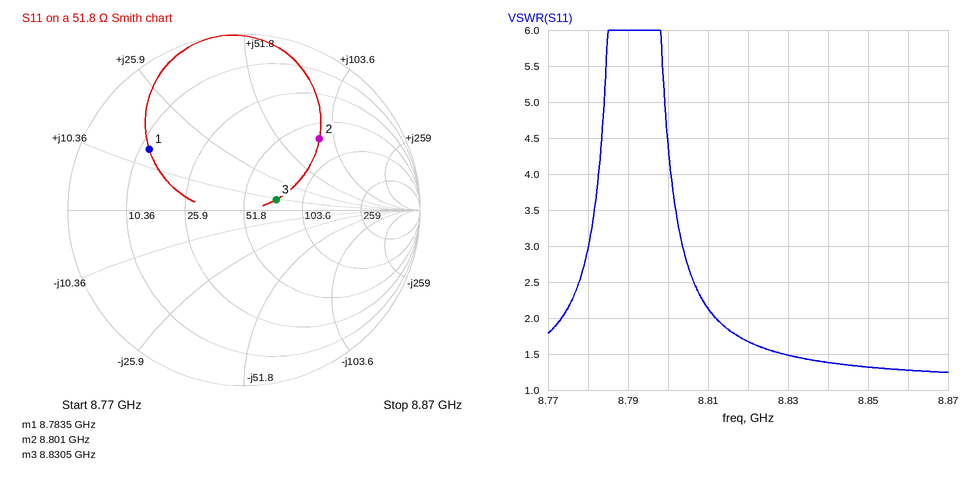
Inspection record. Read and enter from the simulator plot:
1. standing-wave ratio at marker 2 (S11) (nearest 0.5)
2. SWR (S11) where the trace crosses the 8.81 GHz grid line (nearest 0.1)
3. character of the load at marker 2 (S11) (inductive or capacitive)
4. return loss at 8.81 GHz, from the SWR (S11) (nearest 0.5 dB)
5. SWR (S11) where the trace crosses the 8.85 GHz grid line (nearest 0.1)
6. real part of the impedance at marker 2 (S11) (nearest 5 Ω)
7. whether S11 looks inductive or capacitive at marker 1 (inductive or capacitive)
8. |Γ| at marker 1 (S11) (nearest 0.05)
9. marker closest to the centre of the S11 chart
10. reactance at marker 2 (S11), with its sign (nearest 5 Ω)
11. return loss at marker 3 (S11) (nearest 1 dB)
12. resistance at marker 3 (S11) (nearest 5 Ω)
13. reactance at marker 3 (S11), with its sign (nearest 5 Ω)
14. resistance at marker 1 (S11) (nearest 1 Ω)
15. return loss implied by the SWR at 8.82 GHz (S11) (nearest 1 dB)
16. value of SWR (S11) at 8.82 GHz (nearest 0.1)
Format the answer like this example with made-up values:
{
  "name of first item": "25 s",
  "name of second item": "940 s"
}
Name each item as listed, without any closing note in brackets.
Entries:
{
  "standing-wave ratio at marker 2 (S11)": "4.0",
  "SWR (S11) where the trace crosses the 8.81 GHz grid line": "2.1",
  "character of the load at marker 2 (S11)": "inductive",
  "return loss at 8.81 GHz, from the SWR (S11)": "9.0 dB",
  "SWR (S11) where the trace crosses the 8.85 GHz grid line": "1.3",
  "real part of the impedance at marker 2 (S11)": "70 Ω",
  "whether S11 looks inductive or capacitive at marker 1": "inductive",
  "|Γ| at marker 1 (S11)": "0.65",
  "marker closest to the centre of the S11 chart": "marker 3",
  "reactance at marker 2 (S11), with its sign": "+85 Ω",
  "return loss at marker 3 (S11)": "14 dB",
  "resistance at marker 3 (S11)": "75 Ω",
  "reactance at marker 3 (S11), with its sign": "+10 Ω",
  "resistance at marker 1 (S11)": "12 Ω",
  "return loss implied by the SWR at 8.82 GHz (S11)": "12 dB",
  "value of SWR (S11) at 8.82 GHz": "1.7"
}
